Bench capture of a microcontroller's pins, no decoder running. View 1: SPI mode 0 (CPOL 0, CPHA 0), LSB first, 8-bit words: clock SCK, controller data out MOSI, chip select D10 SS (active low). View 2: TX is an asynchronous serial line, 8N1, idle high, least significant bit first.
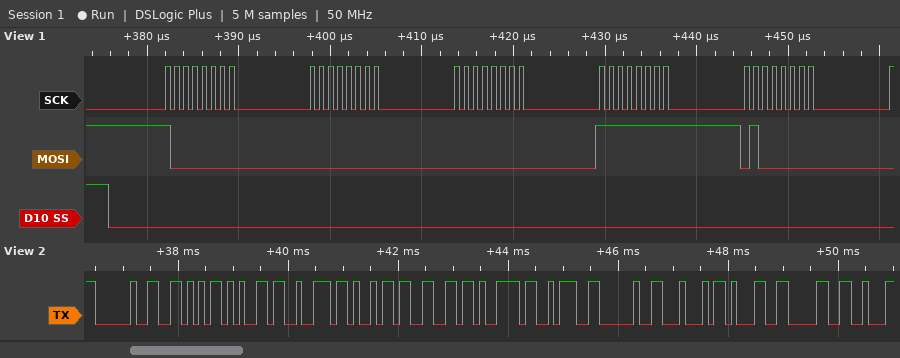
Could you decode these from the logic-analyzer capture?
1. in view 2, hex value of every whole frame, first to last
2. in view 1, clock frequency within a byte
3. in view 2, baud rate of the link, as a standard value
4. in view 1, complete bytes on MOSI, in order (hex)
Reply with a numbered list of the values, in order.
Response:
1. 20 56 65 72 69 66 79 3A 20 44 31 30
2. 1 MHz
3. 9600 baud
4. 01 00 00 FF 02
